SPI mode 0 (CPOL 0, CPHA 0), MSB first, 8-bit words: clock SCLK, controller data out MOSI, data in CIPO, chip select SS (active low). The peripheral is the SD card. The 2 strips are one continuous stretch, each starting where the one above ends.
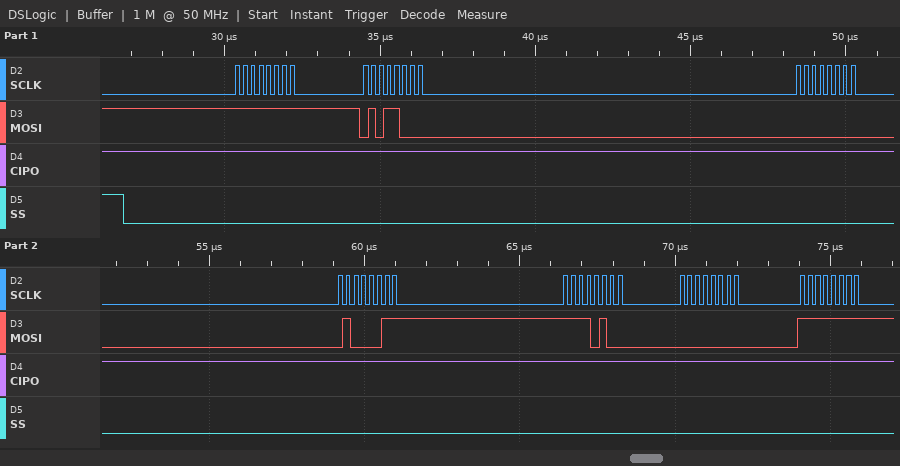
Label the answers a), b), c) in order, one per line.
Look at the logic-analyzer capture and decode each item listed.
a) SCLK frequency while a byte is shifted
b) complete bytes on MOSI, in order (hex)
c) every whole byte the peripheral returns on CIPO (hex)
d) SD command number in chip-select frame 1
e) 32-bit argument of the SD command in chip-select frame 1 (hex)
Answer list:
a) 4 MHz
b) FF 58 00 43 F4 00 FF
c) FF FF FF FF FF FF FF
d) CMD24
e) 0x0043F400
